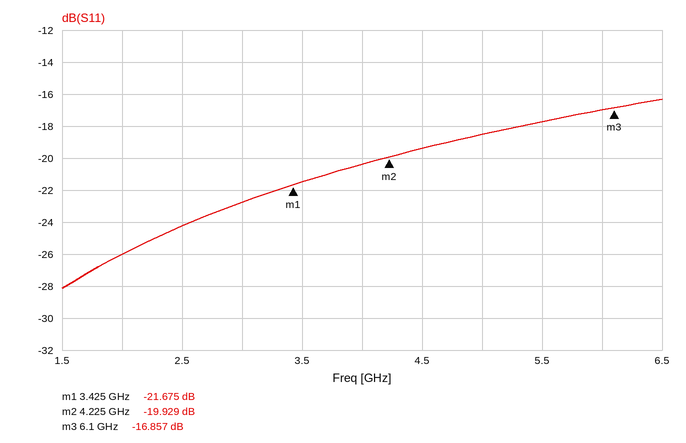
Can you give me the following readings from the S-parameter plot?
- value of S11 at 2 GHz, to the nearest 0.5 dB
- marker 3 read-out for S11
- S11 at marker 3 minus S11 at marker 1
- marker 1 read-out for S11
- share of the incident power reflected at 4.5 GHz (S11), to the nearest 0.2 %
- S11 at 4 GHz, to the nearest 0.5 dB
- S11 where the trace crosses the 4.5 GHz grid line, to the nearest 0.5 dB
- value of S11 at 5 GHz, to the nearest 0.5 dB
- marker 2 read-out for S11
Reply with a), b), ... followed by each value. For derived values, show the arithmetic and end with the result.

a) -26.0 dB
b) -16.857 dB
c) -16.857 − (-21.675) = 4.818 dB
d) -21.675 dB
e) 10^(-19.5/10) ≈ 1.12 %, so 1.2 % to the nearest 0.2 %
f) -20.5 dB
g) -19.5 dB
h) -18.5 dB
i) -19.929 dB
